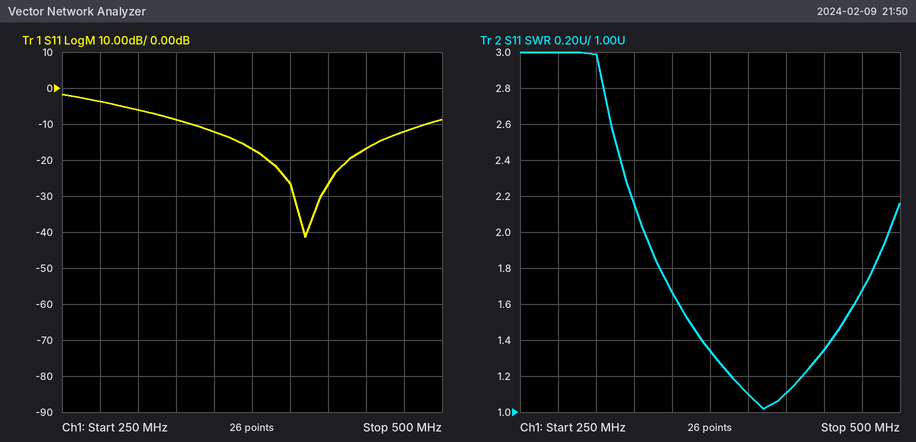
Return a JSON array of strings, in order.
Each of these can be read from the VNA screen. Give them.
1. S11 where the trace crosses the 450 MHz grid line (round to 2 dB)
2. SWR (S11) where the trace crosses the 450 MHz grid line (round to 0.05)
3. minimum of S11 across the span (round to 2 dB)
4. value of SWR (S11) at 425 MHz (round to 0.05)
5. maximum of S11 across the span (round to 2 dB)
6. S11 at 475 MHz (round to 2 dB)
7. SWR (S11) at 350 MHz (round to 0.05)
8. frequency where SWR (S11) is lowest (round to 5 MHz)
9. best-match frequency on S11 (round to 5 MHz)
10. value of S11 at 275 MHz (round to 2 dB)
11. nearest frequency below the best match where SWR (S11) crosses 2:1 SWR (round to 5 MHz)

["-16 dB", "1.35", "-42 dB", "1.10", "-2 dB", "-12 dB", "1.65", "410 MHz", "410 MHz", "-4 dB", "330 MHz"]
